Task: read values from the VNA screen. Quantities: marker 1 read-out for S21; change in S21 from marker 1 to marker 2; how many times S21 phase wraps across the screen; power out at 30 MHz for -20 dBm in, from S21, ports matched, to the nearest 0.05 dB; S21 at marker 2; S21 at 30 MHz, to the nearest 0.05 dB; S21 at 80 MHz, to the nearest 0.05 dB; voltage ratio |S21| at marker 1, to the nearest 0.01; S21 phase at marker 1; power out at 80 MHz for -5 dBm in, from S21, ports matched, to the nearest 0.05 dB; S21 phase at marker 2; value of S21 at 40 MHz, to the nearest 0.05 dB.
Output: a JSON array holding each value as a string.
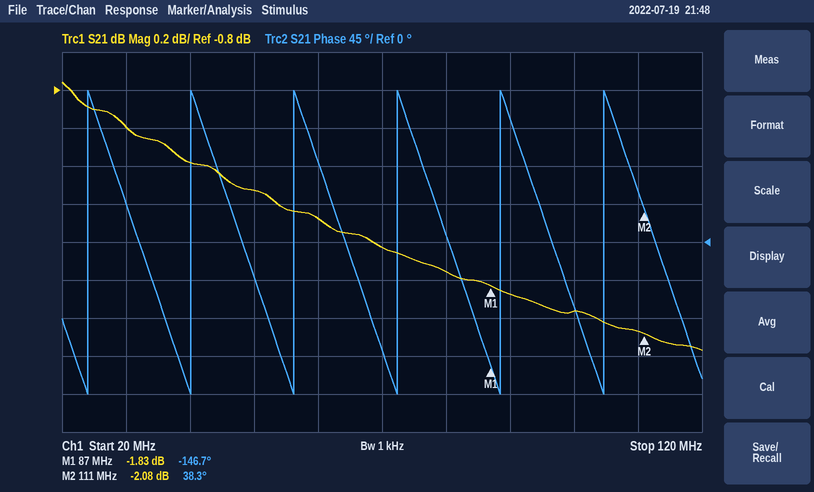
["-1.83 dB", "-0.25 dB", "6", "-21.00 dBm", "-2.08 dB", "-1.00 dB", "-1.75 dB", "0.81", "-146.7°", "-6.75 dBm", "38.3°", "-1.20 dB"]
